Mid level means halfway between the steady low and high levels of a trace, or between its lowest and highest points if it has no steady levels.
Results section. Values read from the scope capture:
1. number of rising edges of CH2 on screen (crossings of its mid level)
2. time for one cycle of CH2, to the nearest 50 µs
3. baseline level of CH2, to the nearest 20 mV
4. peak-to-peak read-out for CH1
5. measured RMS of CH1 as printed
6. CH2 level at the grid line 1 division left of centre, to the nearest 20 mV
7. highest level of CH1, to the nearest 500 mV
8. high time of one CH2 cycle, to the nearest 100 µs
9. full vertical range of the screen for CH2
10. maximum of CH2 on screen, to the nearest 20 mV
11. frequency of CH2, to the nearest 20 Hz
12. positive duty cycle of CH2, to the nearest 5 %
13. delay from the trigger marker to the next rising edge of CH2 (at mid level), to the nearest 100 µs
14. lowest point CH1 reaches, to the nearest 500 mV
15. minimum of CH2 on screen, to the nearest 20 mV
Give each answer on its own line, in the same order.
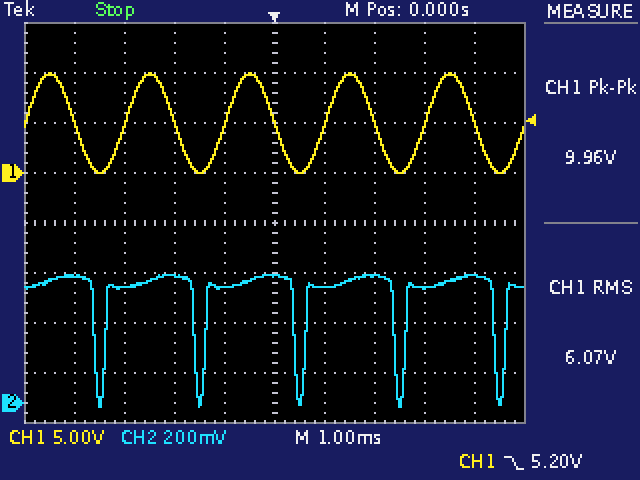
5
2.00 ms
480 mV
9.96 V
6.07 V
460 mV
10.0 V
1.8 ms
1.6 V
520 mV
500 Hz
90 %
600 µs
0.0 V
-20 mV
